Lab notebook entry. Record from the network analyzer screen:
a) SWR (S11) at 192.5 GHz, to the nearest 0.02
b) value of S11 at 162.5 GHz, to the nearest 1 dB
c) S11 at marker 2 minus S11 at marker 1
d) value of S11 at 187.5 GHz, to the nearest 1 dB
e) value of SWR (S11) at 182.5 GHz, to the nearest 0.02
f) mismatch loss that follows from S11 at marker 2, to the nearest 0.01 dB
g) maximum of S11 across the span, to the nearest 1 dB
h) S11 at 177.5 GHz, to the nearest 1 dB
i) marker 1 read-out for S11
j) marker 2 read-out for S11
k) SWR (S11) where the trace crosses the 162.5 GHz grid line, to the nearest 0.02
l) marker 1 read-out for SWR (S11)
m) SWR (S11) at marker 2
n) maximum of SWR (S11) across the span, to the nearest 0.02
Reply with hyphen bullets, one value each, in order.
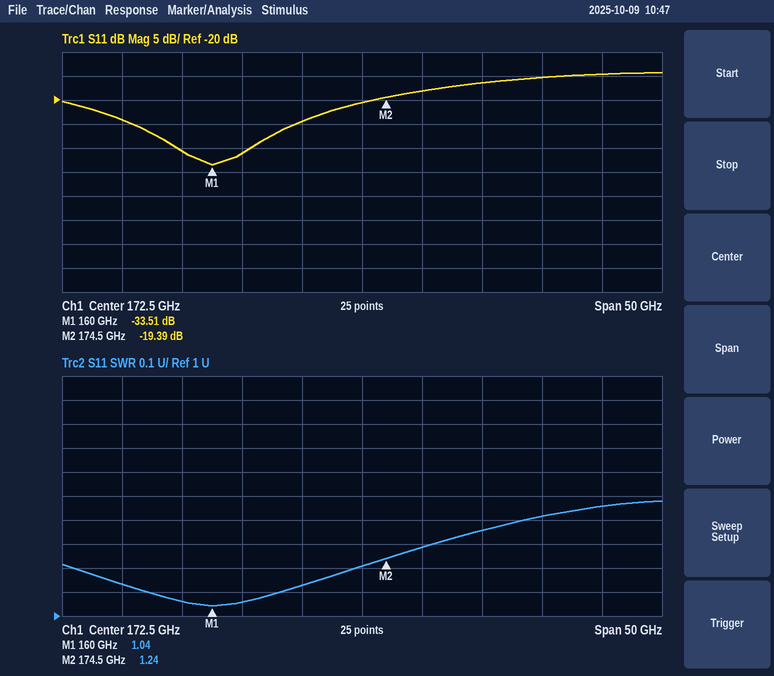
- 1.46
- -31 dB
- 14.12 dB
- -15 dB
- 1.36
- 0.05 dB
- -14 dB
- -18 dB
- -33.51 dB
- -19.39 dB
- 1.06
- 1.04
- 1.24
- 1.48
